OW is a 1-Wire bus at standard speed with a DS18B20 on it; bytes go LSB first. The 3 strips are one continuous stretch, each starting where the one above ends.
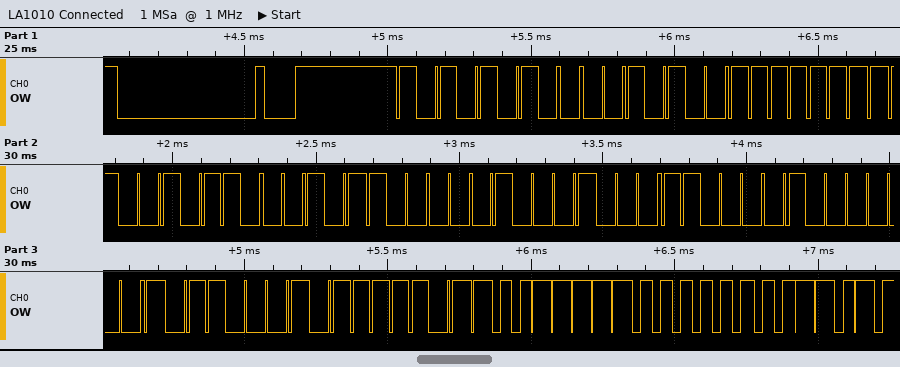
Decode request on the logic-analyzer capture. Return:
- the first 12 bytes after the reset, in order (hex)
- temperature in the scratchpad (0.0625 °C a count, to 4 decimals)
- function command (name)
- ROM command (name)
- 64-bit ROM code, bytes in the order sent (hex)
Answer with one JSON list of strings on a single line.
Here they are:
["55 28 FF 69 34 88 18 02 8D BE F9 00", "15.5625 °C", "Read Scratchpad", "Match ROM", "28 FF 69 34 88 18 02 8D"]
